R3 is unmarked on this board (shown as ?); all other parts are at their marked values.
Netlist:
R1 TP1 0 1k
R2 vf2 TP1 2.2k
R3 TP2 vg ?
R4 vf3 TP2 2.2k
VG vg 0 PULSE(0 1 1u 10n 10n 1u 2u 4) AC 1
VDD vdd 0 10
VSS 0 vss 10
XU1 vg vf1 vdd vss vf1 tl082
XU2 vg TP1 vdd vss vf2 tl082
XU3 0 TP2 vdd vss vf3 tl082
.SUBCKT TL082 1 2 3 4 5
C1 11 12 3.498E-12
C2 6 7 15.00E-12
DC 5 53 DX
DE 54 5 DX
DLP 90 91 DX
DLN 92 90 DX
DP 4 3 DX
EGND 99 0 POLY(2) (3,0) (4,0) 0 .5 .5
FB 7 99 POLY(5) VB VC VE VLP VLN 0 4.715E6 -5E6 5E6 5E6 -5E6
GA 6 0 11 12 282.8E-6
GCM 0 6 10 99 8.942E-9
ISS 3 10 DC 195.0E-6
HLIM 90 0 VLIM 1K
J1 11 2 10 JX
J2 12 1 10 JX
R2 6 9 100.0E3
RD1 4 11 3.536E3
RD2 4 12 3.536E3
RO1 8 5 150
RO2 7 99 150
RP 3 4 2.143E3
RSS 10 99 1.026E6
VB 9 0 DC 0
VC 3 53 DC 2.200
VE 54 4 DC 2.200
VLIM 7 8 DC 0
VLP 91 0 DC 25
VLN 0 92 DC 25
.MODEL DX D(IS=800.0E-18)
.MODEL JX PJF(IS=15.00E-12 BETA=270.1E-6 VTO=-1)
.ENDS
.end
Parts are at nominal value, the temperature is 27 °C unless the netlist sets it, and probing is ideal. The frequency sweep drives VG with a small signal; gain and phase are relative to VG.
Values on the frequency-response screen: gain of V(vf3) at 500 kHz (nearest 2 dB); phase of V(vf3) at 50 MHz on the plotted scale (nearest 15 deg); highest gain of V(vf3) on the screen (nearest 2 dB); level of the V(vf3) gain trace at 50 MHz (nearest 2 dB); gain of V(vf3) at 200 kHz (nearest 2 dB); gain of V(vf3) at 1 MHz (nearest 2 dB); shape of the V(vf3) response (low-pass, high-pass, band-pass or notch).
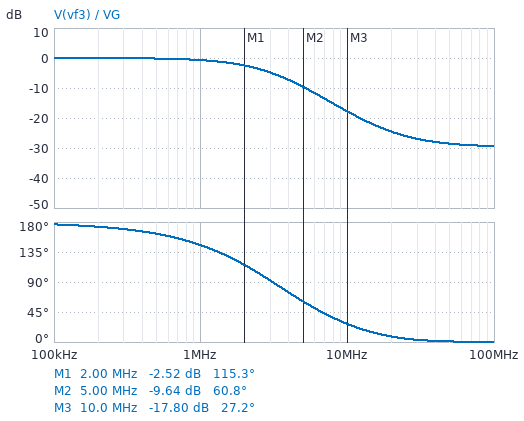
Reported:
0 dB
0 deg
0 dB
-28 dB
0 dB
0 dB
low-pass
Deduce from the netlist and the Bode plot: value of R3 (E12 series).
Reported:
2.2 kΩ
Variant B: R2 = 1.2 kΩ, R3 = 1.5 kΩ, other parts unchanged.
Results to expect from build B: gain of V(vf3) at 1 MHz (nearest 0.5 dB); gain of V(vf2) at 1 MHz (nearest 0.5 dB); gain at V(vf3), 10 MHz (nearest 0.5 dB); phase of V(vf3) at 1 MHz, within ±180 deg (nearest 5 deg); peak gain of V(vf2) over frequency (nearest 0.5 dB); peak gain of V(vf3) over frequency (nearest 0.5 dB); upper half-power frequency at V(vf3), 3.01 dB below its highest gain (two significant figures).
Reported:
2.0 dB
6.0 dB
-16.5 dB
140 deg
7.0 dB
3.5 dB
1.7 MHz
